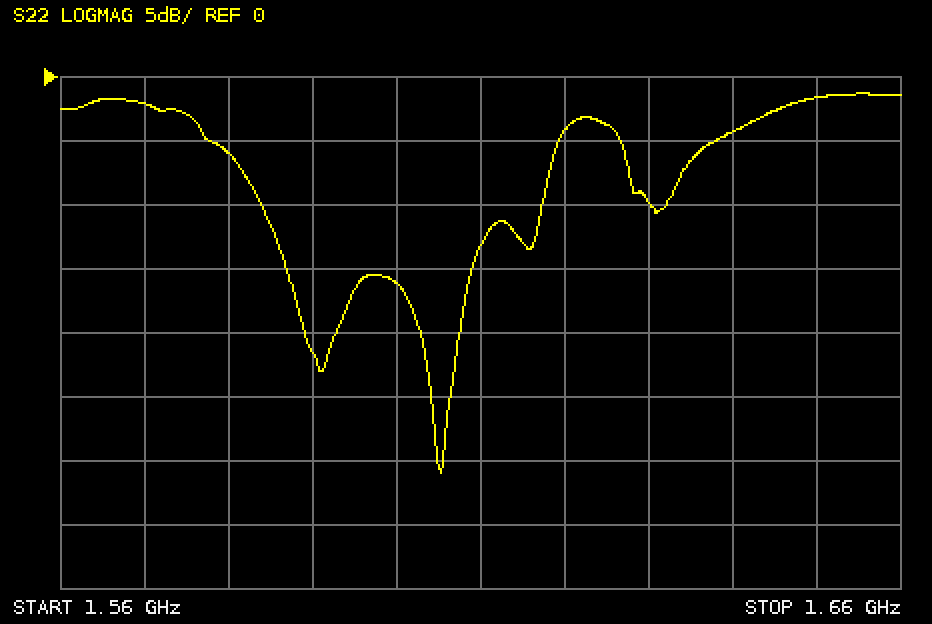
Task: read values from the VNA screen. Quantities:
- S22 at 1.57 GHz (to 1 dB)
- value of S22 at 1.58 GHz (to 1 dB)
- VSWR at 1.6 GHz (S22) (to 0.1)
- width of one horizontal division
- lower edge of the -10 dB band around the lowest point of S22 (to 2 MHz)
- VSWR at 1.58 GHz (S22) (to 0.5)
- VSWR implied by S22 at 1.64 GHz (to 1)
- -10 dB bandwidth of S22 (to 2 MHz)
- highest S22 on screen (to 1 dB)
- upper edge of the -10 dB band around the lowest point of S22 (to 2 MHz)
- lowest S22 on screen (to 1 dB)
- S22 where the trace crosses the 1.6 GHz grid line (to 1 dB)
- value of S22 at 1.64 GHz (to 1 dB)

-2 dB
-6 dB
1.4
10 MHz
1.584 GHz
3.0
4
34 MHz
-1 dB
1.618 GHz
-31 dB
-16 dB
-4 dB
